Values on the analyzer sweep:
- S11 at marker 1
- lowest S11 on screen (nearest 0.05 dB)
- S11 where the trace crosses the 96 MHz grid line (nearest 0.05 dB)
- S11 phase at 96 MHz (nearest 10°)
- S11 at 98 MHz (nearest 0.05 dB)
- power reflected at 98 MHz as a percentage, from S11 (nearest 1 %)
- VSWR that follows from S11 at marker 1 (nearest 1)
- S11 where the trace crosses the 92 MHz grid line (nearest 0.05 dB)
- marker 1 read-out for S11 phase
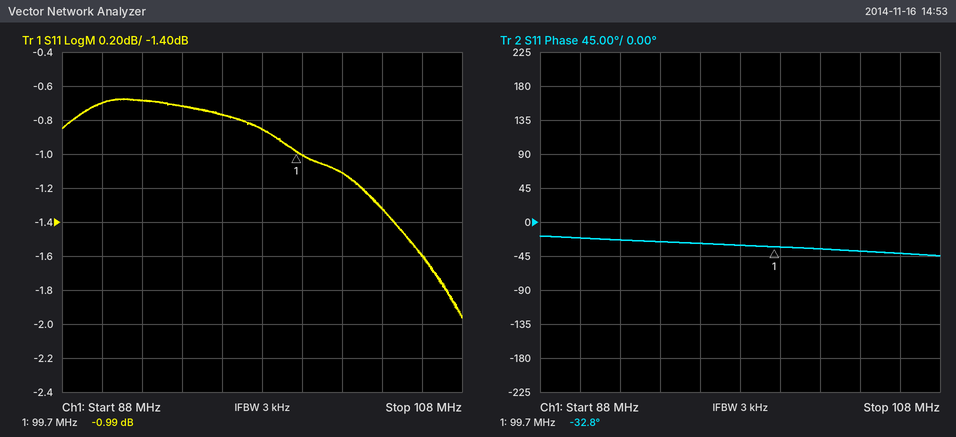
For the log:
-0.99 dB
-1.95 dB
-0.75 dB
-30°
-0.85 dB
82 %
18
-0.70 dB
-32.8°
